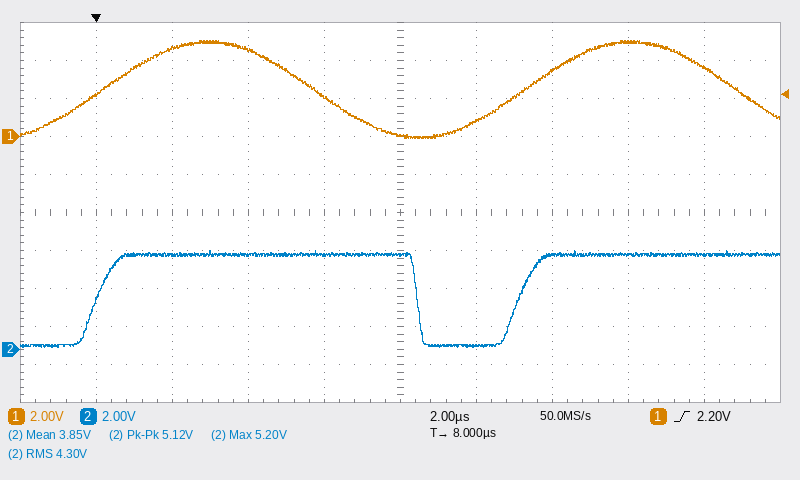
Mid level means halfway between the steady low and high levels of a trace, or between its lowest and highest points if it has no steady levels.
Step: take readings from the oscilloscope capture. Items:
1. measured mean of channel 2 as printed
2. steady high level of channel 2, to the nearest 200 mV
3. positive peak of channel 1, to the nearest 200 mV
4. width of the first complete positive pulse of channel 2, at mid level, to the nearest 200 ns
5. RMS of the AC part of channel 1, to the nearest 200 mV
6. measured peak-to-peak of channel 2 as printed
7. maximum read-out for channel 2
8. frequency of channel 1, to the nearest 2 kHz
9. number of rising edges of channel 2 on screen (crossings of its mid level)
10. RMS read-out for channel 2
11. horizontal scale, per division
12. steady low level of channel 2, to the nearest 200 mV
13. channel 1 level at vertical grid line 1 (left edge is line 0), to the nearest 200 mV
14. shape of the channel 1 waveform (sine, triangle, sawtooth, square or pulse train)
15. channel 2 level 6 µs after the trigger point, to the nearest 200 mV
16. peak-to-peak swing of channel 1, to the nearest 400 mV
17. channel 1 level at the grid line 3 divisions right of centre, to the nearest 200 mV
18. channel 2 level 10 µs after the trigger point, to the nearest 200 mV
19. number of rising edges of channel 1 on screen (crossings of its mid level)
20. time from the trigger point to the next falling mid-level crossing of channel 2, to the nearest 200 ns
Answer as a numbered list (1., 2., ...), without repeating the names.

1. 3.85 V
2. 5.0 V
3. 5.0 V
4. 8.4 µs
5. 1.8 V
6. 5.12 V
7. 5.20 V
8. 90 kHz
9. 2
10. 4.30 V
11. 2 µs
12. 200 mV
13. 2.2 V
14. sine
15. 5.0 V
16. 5.2 V
17. 5.0 V
18. 200 mV
19. 2
20. 8.4 µs
